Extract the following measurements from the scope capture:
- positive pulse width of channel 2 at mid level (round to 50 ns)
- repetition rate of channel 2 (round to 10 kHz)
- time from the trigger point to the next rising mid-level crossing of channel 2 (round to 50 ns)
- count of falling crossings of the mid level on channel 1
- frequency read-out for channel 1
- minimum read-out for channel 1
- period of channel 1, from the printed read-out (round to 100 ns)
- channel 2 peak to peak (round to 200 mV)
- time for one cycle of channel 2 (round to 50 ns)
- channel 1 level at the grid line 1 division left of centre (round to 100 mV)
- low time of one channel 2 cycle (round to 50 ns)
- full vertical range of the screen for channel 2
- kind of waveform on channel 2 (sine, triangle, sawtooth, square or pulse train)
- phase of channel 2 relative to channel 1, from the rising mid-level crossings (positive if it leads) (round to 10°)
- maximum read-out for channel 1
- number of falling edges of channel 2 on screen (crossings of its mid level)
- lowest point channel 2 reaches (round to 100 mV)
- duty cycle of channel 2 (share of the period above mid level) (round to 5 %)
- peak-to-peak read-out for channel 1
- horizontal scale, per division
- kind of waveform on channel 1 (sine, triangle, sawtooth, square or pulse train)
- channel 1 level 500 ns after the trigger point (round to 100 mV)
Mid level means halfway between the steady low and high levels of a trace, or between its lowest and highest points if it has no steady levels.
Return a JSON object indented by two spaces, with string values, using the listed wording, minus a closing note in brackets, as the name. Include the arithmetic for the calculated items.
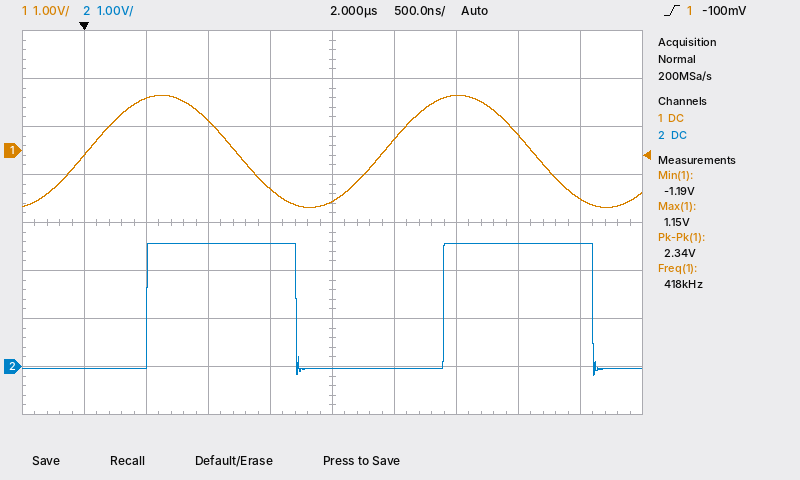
{
  "positive pulse width of channel 2 at mid level": "1.20 µs",
  "repetition rate of channel 2": "1 / 2.40 µs ≈ 417 kHz, so 420 kHz to the nearest 10 kHz",
  "time from the trigger point to the next rising mid-level crossing of channel 2": "500 ns",
  "count of falling crossings of the mid level on channel 1": "2",
  "frequency read-out for channel 1": "418 kHz",
  "minimum read-out for channel 1": "-1.19 V",
  "period of channel 1, from the printed read-out": "1 / 418 kHz ≈ 2.4 µs",
  "channel 2 peak to peak": "2.8 V",
  "time for one cycle of channel 2": "2.40 µs",
  "channel 1 level at the grid line 1 division left of centre": "-800 mV",
  "low time of one channel 2 cycle": "1.20 µs",
  "full vertical range of the screen for channel 2": "8 V",
  "kind of waveform on channel 2": "square",
  "phase of channel 2 relative to channel 1, from the rising mid-level crossings (positive if it leads)": "-70°",
  "maximum read-out for channel 1": "1.15 V",
  "number of falling edges of channel 2 on screen": "2",
  "lowest point channel 2 reaches": "-200 mV",
  "duty cycle of channel 2 (share of the period above mid level)": "1.20 µs / 2.40 µs ≈ 50 %",
  "peak-to-peak read-out for channel 1": "2.34 V",
  "horizontal scale, per division": "500 ns",
  "kind of waveform on channel 1": "sine",
  "channel 1 level 500 ns after the trigger point": "1.1 V"
}
